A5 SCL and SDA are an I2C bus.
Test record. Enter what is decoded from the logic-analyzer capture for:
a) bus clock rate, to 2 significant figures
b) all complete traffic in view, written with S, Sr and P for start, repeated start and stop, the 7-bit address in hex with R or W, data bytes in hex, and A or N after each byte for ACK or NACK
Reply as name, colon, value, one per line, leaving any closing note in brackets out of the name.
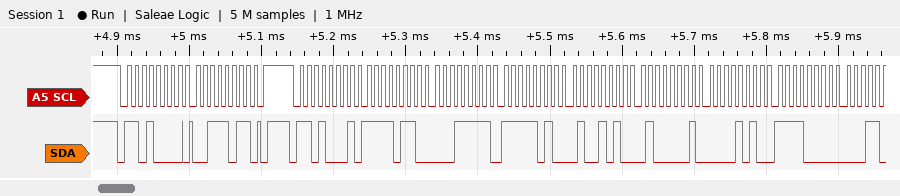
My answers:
bus clock rate, to 2 significant figures: 100 kHz
all complete traffic in view, written with S, Sr and P for start, repeated start and stop, the 7-bit address in hex with R or W, data bytes in hex, and A or N after each byte for ACK or NACK: S 68W A 3B A P S 68R A F6 A 1F A FA A 4A A 41 A 0A A F0 A
